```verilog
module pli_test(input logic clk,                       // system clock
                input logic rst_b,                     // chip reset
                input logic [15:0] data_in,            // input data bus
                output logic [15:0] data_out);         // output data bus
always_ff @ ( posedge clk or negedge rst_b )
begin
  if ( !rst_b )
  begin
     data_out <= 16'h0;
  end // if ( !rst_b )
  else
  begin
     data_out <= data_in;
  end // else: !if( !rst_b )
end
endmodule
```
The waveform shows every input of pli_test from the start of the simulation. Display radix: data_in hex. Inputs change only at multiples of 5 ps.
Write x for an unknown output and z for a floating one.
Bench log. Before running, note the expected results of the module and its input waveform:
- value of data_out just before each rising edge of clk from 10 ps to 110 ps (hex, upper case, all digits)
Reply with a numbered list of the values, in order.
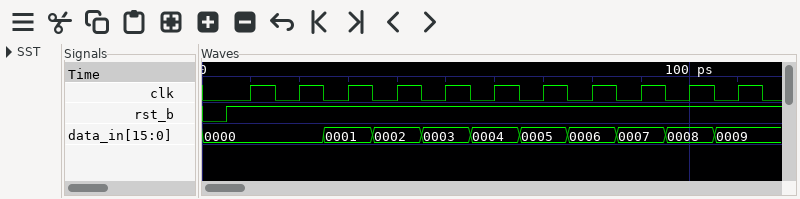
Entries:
1. 0000, 0000, 0000, 0001, 0002, 0003, 0004, 0005, 0006, 0007, 0008
